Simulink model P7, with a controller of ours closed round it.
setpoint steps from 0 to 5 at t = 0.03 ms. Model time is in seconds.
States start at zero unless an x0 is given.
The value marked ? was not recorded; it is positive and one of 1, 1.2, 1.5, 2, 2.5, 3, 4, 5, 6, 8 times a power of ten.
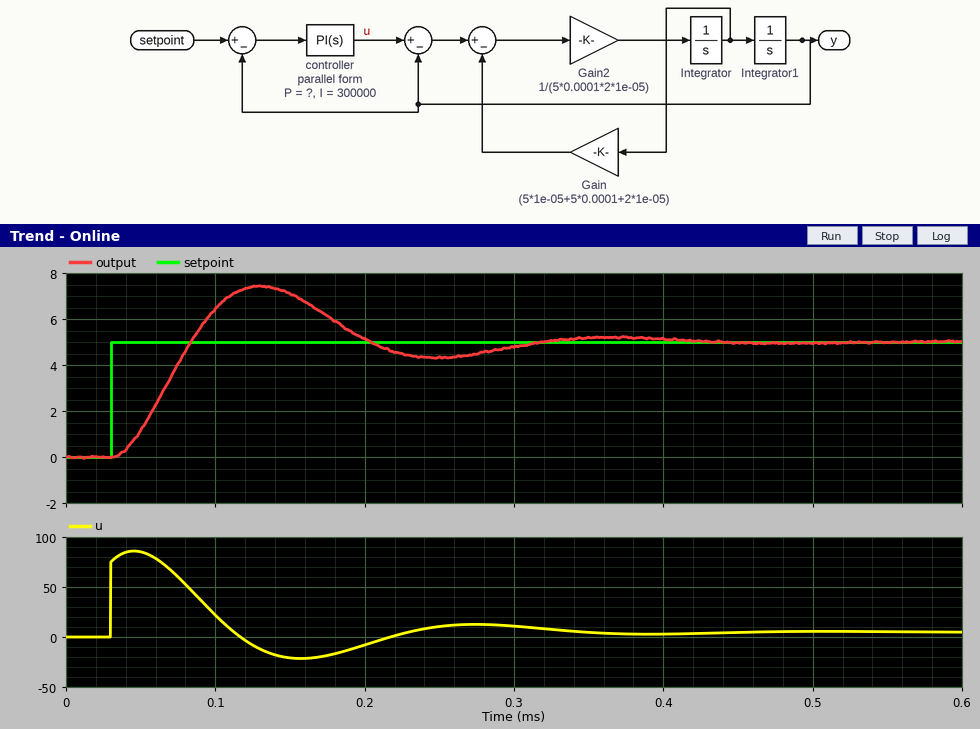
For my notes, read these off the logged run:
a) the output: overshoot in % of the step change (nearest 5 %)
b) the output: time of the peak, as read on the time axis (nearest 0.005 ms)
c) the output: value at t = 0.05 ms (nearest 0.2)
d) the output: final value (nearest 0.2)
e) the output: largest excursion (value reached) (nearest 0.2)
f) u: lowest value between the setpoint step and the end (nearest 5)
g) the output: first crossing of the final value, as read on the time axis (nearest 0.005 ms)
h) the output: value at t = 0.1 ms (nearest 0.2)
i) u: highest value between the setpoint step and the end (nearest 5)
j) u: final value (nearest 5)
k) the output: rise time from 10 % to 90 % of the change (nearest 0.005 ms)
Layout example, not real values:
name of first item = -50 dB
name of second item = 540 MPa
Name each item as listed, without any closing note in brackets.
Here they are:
the output: overshoot in % of the step change = 50 %
the output: time of the peak, as read on the time axis = 0.130 ms
the output: value at t = 0.05 ms = 1.2
the output: final value = 5.0
the output: largest excursion (value reached) = 7.4
u: lowest value between the setpoint step and the end = -20
the output: first crossing of the final value, as read on the time axis = 0.085 ms
the output: value at t = 0.1 ms = 6.4
u: highest value between the setpoint step and the end = 85
u: final value = 5
the output: rise time from 10 % to 90 % of the change = 0.035 ms
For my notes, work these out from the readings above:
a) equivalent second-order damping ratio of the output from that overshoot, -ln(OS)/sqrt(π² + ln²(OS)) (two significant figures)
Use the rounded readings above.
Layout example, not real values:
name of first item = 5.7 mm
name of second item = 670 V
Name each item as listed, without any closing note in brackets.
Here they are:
equivalent second-order damping ratio of the output from that overshoot, -ln(OS)/sqrt(π² + ln²(OS)) = 0.22
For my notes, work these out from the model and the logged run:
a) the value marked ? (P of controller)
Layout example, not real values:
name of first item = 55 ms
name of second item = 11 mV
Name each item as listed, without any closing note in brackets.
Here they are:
the value marked ? = 15
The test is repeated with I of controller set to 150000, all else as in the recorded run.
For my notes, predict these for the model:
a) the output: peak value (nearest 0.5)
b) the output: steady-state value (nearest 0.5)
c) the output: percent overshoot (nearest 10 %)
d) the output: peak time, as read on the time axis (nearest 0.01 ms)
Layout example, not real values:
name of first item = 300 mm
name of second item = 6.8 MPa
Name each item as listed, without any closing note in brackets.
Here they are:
the output: peak value = 6.5
the output: steady-state value = 5.0
the output: percent overshoot = 30 %
the output: peak time, as read on the time axis = 0.14 ms
